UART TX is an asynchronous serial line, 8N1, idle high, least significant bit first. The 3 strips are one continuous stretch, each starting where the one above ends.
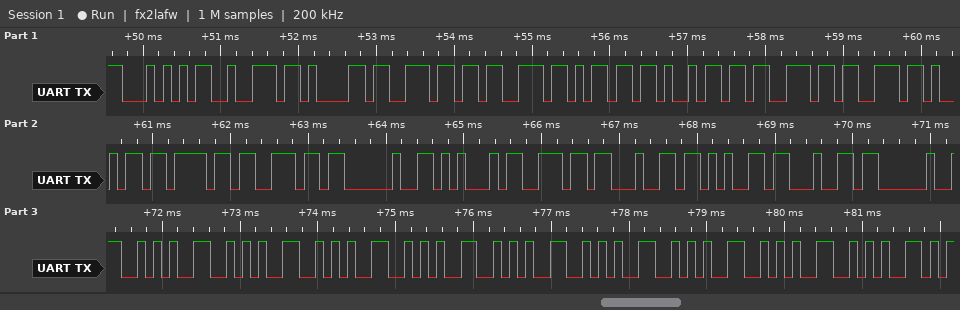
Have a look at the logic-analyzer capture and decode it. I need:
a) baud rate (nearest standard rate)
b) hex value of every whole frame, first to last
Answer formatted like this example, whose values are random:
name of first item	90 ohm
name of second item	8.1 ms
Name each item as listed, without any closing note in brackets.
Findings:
baud rate	9600 baud
hex value of every whole frame, first to last	0x54 0x72 0x61 0x6E 0x73 0x6D 0x69 0x73 0x73 0x69 0x6F 0x6E 0x20 0x45 0x6E 0x64 0x65 0x64 0x20 0x2A 0x2A 0x2A 0x2A 0x2A 0x2A 0x2A 0x2A 0x2A
